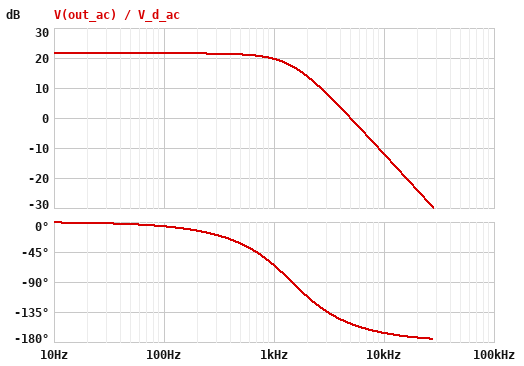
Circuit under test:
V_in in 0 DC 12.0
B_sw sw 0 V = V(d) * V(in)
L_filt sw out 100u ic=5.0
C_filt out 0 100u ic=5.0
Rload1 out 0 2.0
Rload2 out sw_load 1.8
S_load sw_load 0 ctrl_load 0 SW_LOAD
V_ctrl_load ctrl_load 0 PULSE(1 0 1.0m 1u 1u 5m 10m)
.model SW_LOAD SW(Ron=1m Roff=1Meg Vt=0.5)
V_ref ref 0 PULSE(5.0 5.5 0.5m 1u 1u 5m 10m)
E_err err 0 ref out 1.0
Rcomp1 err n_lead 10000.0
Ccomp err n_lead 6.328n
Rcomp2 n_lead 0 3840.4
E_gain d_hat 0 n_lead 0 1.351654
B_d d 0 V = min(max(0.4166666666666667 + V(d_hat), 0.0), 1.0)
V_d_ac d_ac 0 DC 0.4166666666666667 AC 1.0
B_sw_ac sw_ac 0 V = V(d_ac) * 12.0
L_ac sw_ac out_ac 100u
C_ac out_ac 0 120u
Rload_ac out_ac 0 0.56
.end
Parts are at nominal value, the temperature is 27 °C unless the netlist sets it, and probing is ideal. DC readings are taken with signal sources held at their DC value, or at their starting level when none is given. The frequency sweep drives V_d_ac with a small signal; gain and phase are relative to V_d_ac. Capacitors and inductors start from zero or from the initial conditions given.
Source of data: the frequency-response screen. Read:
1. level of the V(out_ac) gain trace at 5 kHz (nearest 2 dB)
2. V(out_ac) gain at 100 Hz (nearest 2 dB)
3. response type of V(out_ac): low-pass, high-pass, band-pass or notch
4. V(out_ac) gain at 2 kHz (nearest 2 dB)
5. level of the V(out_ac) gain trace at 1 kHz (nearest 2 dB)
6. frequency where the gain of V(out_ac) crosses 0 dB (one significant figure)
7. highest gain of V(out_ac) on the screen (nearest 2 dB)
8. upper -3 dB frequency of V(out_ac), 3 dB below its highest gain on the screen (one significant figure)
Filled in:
0 dB
22 dB
low-pass
14 dB
20 dB
5 kHz
22 dB
1 kHz
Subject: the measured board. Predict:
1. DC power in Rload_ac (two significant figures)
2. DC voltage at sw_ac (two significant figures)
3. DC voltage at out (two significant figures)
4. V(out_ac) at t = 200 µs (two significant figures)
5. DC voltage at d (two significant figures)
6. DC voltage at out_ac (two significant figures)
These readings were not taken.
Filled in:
45 W
5.0 V
5.0 V
3.1 V
420 mV
5.0 V
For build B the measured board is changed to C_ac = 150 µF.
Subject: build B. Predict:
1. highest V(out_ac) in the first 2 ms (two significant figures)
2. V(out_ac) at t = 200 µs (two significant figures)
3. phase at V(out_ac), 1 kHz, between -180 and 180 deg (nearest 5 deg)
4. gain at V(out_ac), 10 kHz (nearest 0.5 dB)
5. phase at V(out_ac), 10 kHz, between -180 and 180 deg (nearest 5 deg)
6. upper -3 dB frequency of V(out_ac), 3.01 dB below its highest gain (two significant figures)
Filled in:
5.2 V
2.9 V
-70 deg
-14.0 dB
-170 deg
1.3 kHz
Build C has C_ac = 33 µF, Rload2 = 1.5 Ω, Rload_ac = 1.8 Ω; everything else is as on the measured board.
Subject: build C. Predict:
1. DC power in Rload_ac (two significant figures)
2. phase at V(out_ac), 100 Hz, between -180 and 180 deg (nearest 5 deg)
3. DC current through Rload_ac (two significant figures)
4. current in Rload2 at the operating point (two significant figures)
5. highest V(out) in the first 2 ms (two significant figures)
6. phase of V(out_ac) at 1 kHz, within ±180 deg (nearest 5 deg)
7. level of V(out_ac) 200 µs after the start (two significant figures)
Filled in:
14 W
0 deg
2.8 A
3.3 A
6.5 V
-20 deg
5.9 V
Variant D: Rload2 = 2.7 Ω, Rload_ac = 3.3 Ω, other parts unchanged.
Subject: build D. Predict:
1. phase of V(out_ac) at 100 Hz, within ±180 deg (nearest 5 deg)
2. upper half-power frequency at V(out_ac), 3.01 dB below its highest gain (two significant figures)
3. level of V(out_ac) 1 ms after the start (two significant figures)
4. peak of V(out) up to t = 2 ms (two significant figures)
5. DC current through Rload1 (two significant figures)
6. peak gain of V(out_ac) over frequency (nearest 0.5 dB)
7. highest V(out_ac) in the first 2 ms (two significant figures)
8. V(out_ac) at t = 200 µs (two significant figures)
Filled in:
0 deg
1.6 kHz
6.2 V
5.9 V
2.5 A
33.0 dB
8.2 V
5.4 V
